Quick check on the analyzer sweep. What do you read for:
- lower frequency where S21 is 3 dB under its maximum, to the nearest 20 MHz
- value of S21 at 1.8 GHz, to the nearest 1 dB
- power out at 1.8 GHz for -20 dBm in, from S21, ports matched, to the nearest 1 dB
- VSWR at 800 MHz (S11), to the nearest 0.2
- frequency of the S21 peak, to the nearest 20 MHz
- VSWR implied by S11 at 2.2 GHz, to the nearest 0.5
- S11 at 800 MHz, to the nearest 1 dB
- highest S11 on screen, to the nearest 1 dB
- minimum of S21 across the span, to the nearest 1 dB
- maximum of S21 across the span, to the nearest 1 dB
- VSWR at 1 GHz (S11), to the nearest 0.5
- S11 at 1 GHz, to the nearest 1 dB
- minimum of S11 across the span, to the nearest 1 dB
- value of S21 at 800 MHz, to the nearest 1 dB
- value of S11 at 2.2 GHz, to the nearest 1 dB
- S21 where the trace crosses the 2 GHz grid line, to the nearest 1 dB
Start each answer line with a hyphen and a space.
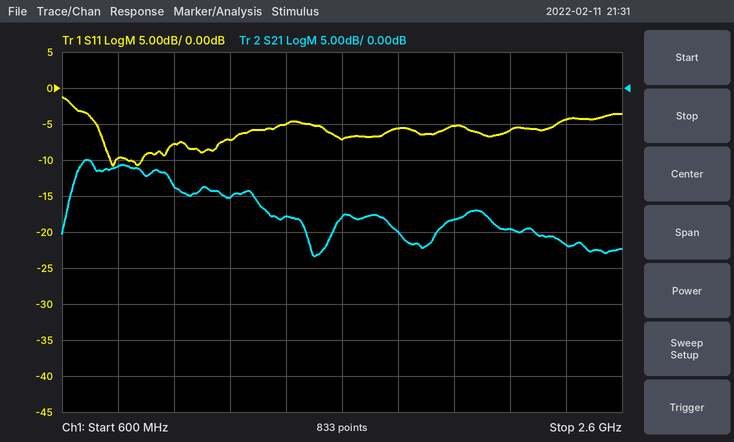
- 640 MHz
- -20 dB
- -40 dBm
- 2.0
- 680 MHz
- 3.0
- -10 dB
- -1 dB
- -23 dB
- -10 dB
- 2.5
- -8 dB
- -11 dB
- -11 dB
- -6 dB
- -18 dB
